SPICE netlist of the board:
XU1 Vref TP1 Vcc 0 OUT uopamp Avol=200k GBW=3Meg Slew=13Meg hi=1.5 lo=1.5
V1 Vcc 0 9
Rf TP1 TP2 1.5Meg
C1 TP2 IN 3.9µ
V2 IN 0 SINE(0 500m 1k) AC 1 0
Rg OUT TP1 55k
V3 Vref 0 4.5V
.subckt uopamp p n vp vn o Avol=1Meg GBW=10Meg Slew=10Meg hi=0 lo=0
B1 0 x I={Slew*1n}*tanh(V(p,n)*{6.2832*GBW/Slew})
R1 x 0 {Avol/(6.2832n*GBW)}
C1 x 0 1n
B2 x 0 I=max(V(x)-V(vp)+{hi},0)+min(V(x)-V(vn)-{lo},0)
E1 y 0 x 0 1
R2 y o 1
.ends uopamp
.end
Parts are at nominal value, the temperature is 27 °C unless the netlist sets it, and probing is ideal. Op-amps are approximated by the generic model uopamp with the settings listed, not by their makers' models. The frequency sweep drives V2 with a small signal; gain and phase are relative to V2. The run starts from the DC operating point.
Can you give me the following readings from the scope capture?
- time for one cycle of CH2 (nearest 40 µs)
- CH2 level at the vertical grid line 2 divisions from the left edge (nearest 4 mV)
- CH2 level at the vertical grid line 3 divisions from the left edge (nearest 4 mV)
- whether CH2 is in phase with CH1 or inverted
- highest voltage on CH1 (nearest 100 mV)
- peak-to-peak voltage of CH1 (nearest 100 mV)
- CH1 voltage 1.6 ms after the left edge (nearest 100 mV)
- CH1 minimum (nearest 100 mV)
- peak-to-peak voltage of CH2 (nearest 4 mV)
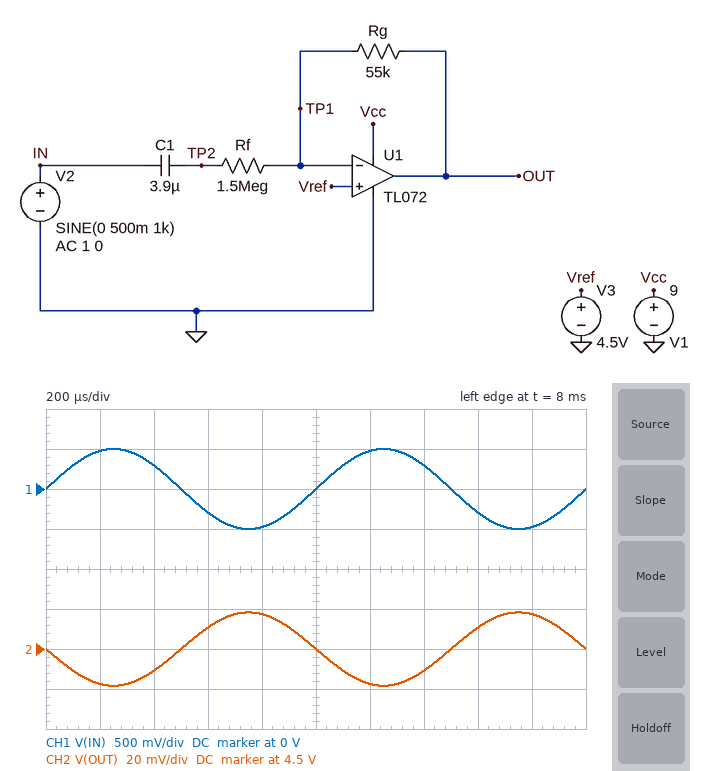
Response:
1.00 ms
4.488 V
4.512 V
inverted
500 mV
1.0 V
-300 mV
-500 mV
36 mV
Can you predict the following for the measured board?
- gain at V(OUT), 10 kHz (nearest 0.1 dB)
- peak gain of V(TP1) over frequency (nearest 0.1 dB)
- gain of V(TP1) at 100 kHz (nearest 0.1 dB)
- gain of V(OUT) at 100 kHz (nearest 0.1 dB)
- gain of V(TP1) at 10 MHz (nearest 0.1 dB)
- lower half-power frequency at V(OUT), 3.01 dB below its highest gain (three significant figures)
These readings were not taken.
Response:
-28.7 dB
-29.0 dB
-58.3 dB
-28.7 dB
-29.4 dB
27.2 mHz
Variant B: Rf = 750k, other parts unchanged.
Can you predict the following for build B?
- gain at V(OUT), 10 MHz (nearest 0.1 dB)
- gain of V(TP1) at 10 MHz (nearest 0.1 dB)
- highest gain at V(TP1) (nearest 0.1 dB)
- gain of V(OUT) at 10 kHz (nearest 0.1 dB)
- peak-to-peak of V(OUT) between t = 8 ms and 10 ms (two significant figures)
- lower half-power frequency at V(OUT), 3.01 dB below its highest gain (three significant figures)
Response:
-34.1 dB
-23.6 dB
-23.3 dB
-22.7 dB
73 mV
54.4 mHz
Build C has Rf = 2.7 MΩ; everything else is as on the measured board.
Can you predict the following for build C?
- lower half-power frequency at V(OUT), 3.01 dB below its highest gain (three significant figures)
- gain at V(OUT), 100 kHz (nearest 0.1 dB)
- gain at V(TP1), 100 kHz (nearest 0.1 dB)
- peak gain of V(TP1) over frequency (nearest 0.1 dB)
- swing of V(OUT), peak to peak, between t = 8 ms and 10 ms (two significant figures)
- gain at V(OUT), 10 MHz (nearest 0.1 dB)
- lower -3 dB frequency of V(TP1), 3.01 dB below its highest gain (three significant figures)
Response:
15.1 mHz
-33.8 dB
-63.4 dB
-34.0 dB
20 mV
-44.8 dB
2.94 MHz
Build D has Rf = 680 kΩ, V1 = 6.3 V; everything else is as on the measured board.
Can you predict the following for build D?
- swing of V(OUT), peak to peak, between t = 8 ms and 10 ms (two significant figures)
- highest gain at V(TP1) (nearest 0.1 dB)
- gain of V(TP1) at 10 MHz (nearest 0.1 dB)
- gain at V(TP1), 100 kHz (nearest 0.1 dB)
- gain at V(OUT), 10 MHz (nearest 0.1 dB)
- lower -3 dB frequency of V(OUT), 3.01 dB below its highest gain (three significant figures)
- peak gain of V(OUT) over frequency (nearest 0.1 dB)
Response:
81 mV
-22.5 dB
-22.8 dB
-51.4 dB
-33.3 dB
60.0 mHz
-21.8 dB
